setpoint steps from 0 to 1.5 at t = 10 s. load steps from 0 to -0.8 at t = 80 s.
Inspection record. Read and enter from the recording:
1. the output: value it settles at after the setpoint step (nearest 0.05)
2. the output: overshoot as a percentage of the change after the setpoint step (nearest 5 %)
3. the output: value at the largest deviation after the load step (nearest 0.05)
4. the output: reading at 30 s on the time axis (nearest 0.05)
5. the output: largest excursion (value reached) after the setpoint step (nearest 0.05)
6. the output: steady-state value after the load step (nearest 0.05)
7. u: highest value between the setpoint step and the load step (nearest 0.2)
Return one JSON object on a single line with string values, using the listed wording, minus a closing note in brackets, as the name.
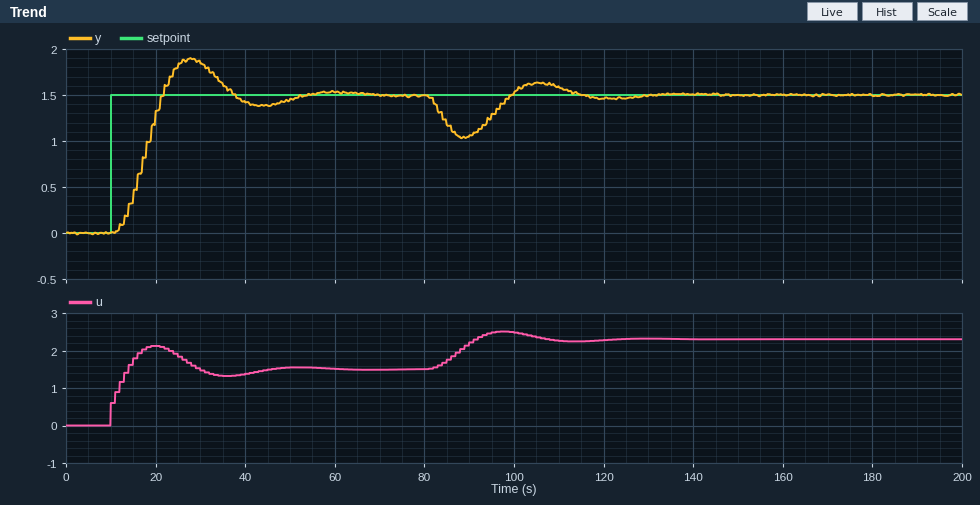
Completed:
{"the output: value it settles at after the setpoint step": "1.50", "the output: overshoot as a percentage of the change after the setpoint step": "25 %", "the output: value at the largest deviation after the load step": "1.05", "the output: reading at 30 s on the time axis": "1.85", "the output: largest excursion (value reached) after the setpoint step": "1.90", "the output: steady-state value after the load step": "1.50", "u: highest value between the setpoint step and the load step": "2.2"}
